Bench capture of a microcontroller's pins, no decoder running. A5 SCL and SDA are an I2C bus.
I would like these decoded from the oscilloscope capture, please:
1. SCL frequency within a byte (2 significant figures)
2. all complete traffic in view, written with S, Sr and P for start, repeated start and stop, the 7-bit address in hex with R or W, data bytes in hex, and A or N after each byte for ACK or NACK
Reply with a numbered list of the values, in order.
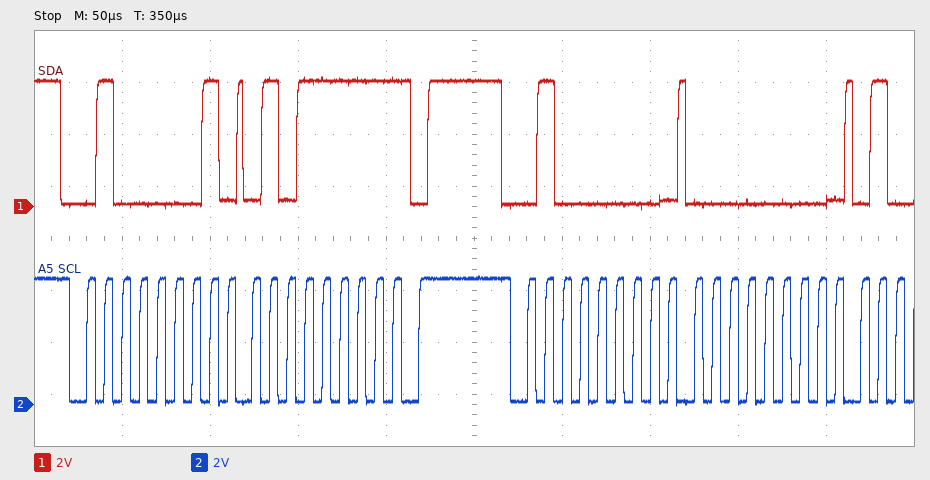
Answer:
1. 100 kHz
2. S 20R A 5F N P S 20W A 00 A
